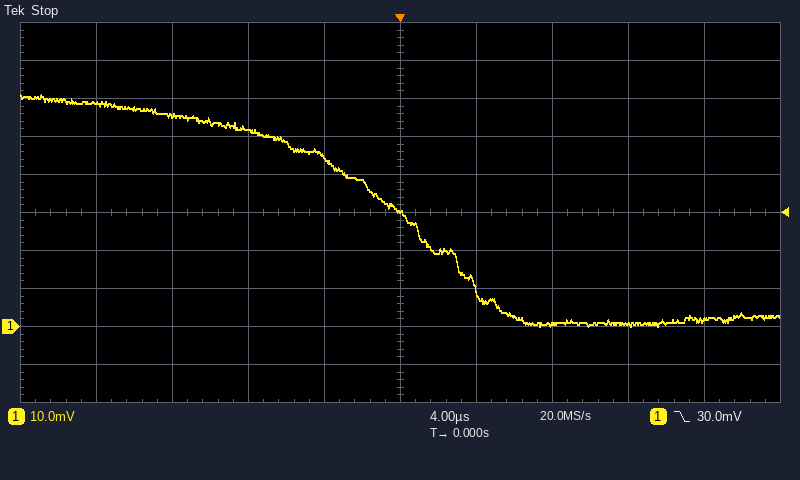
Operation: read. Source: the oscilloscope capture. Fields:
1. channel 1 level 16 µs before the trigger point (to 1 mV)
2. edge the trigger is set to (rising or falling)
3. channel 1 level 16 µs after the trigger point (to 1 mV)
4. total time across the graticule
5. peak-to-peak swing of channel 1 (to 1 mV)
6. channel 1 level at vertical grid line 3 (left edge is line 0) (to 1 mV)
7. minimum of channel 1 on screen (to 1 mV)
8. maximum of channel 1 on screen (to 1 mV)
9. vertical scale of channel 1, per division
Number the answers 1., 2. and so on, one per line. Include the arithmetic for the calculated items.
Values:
1. 59 mV
2. falling
3. 2 mV
4. 40 µs
5. 61 mV − (0 mV) = 61 mV
6. 52 mV
7. 0 mV
8. 61 mV
9. 10 mV
